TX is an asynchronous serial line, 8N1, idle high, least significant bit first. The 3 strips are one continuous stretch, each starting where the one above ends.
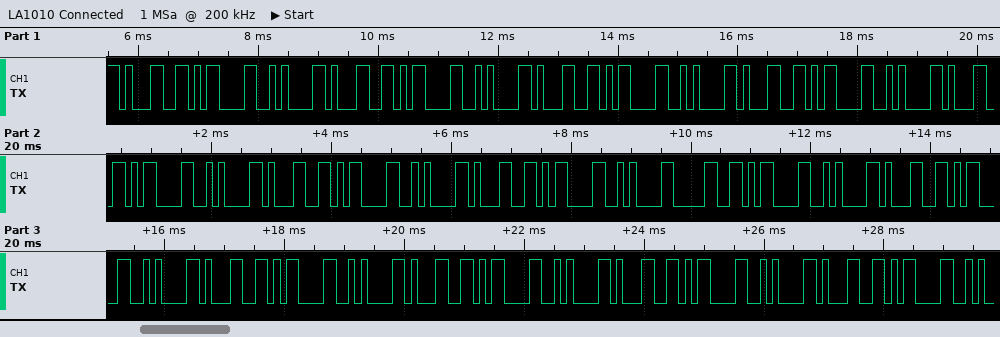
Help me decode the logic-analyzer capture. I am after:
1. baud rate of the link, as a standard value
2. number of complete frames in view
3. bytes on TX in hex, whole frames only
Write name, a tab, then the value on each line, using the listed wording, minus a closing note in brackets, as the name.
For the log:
baud rate of the link, as a standard value	9600 baud
number of complete frames in view	38
bytes on TX in hex, whole frames only	31 0D 0A 31 0D 0A 31 0D 0A 31 0D 0A 31 0D 0A 31 0D 0A 31 0D 0A 30 0D 0A 31 0D 0A 31 0D 0A 31 0D 0A 31 0D 0A 31 0D
